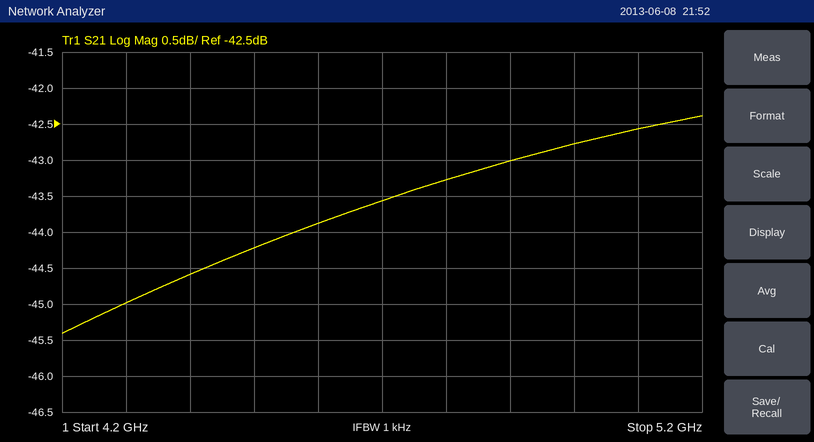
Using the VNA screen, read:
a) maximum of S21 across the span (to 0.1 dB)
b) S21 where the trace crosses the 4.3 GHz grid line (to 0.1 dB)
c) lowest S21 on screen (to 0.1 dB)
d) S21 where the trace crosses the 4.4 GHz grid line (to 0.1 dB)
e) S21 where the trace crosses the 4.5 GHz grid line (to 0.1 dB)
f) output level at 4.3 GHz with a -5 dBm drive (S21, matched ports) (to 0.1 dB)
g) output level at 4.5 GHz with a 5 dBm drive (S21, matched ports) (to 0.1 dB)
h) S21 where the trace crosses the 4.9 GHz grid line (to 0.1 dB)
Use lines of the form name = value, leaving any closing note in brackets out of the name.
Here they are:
maximum of S21 across the span = -42.4 dB
S21 where the trace crosses the 4.3 GHz grid line = -45.0 dB
lowest S21 on screen = -45.4 dB
S21 where the trace crosses the 4.4 GHz grid line = -44.6 dB
S21 where the trace crosses the 4.5 GHz grid line = -44.2 dB
output level at 4.3 GHz with a -5 dBm drive (S21, matched ports) = -50.0 dBm
output level at 4.5 GHz with a 5 dBm drive (S21, matched ports) = -39.2 dBm
S21 where the trace crosses the 4.9 GHz grid line = -43.0 dB
